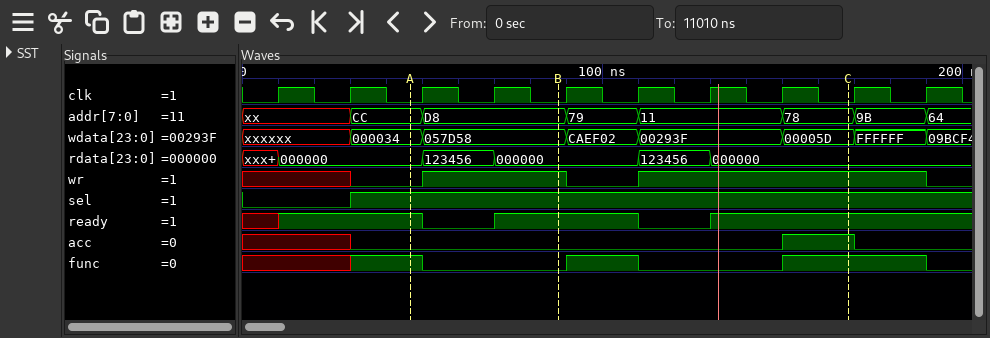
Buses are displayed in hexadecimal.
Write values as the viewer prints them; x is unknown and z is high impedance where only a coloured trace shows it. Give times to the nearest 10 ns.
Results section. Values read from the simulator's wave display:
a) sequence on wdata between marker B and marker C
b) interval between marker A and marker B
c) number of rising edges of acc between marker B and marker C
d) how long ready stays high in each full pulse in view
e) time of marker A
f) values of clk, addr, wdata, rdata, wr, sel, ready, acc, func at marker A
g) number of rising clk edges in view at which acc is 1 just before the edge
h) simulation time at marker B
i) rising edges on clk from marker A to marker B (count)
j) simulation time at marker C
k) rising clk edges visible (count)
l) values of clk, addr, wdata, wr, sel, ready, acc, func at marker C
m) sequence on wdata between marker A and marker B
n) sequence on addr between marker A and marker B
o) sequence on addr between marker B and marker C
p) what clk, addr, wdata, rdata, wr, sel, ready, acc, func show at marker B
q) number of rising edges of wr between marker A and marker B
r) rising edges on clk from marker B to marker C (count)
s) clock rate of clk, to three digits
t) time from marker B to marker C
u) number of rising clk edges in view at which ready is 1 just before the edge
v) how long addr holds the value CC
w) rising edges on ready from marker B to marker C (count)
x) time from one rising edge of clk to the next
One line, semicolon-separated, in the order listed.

057D58, CAEF02, 00293F, 00005D; 40 ns; 1; 40 ns; 50 ns; clk=0, addr=CC, wdata=000034, rdata=000000, wr=0, sel=1, ready=1, acc=0, func=1; 1; 90 ns; 2; 170 ns; 10; clk=0, addr=78, wdata=00005D, wr=1, sel=1, ready=1, acc=1, func=1; 000034, 057D58; CC, D8; D8, 79, 11, 78; clk=0, addr=D8, wdata=057D58, rdata=000000, wr=1, sel=1, ready=1, acc=0, func=0; 1; 4; 50.0 MHz; 80 ns; 7; 20 ns; 1; 20 ns
